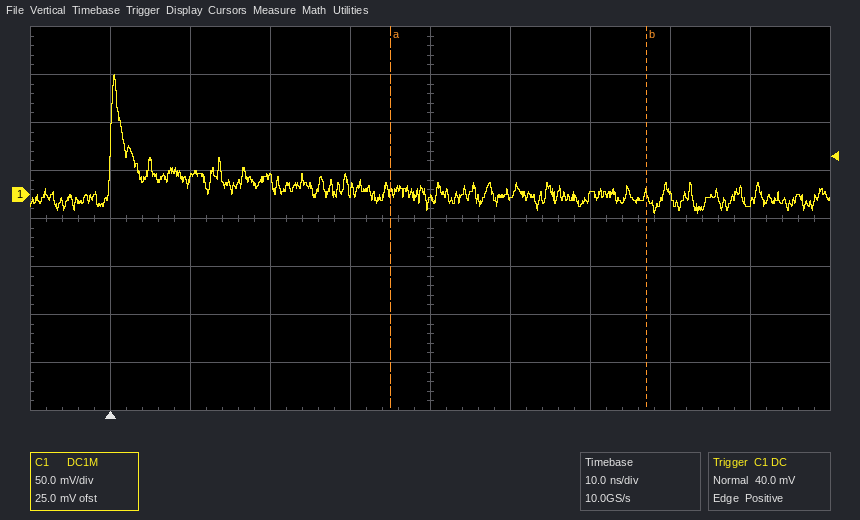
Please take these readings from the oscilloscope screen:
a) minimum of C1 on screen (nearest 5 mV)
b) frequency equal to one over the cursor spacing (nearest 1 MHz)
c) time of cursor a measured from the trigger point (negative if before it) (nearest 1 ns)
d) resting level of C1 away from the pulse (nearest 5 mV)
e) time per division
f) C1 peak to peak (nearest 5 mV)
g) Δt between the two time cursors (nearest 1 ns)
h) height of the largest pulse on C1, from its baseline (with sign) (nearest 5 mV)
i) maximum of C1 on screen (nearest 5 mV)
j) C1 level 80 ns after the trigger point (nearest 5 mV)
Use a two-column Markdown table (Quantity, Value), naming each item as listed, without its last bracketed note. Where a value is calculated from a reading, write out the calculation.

| Quantity | Value |
|---|---|
| minimum of C1 on screen | -20 mV |
| frequency equal to one over the cursor spacing | 1 / 32 ns ≈ 31 MHz |
| time of cursor a measured from the trigger point (negative if before it) | +35 ns |
| resting level of C1 away from the pulse | 0 mV |
| time per division | 10 ns |
| C1 peak to peak | 125 mV − (-20 mV) = 145 mV |
| Δt between the two time cursors | 32 ns |
| height of the largest pulse on C1, from its baseline (with sign) | 125 mV − (0 mV) = +125 mV |
| maximum of C1 on screen | 125 mV |
| C1 level 80 ns after the trigger point | -10 mV |
